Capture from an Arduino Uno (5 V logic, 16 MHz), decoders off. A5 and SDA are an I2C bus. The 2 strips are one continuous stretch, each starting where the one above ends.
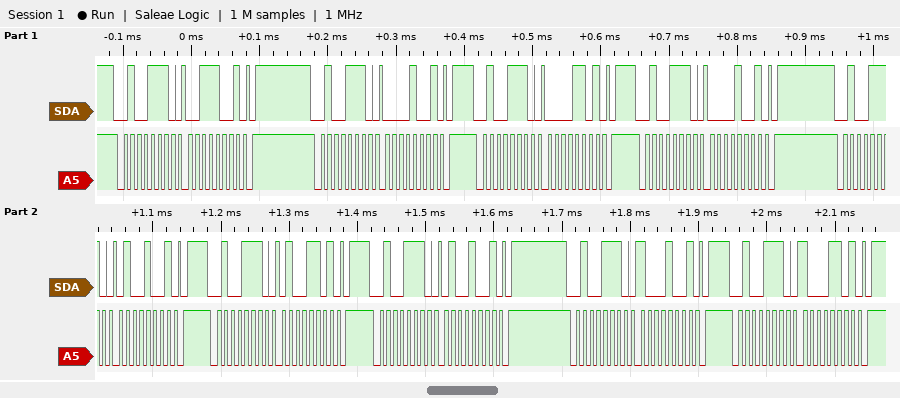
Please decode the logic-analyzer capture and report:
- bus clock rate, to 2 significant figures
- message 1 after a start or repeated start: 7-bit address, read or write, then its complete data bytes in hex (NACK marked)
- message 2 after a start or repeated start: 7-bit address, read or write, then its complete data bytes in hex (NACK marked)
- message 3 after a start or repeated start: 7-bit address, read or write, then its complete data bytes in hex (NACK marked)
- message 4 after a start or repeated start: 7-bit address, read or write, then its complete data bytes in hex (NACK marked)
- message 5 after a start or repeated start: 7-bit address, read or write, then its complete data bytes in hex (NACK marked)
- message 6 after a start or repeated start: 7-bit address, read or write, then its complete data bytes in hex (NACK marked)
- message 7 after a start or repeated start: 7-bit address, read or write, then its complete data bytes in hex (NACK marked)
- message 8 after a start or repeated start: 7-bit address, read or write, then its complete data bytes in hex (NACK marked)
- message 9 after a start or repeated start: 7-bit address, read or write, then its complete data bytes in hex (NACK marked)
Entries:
100 kHz
0x27 write: 39
0x27 write: 09
0x27 write: 0D
0x27 write: 09
0x27 write: 49
0x27 write: 4D
0x27 write: 49
0x27 write: 89
0x27 write: 8D
